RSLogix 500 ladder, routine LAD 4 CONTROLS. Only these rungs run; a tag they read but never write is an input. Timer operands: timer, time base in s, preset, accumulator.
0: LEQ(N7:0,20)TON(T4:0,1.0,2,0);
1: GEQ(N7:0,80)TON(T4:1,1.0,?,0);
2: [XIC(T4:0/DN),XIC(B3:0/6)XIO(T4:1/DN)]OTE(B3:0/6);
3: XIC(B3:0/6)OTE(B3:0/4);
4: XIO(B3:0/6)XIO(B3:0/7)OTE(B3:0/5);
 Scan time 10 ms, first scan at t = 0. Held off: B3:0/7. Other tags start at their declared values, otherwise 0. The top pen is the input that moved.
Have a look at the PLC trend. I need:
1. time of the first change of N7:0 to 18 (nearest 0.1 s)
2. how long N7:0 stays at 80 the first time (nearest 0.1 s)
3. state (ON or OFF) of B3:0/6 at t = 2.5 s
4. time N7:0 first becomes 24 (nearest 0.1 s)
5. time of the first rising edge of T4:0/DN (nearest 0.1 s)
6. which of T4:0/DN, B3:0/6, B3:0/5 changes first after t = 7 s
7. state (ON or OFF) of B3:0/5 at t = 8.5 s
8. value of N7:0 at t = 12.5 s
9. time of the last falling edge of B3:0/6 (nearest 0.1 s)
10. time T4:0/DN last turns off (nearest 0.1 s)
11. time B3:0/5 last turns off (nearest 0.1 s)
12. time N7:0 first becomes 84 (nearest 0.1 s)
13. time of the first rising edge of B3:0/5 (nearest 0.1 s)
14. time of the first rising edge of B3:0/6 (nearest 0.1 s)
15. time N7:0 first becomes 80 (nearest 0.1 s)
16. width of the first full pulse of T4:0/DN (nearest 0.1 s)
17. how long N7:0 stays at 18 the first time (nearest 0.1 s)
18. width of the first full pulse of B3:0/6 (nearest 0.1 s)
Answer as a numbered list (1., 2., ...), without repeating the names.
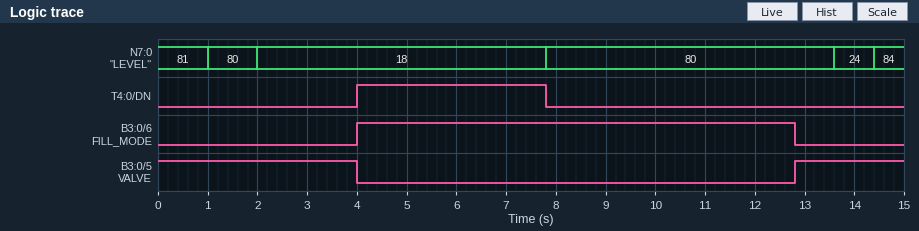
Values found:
1. 2.0 s
2. 1.0 s
3. OFF
4. 13.6 s
5. 4.0 s
6. T4:0/DN
7. OFF
8. 80
9. 12.8 s
10. 7.8 s
11. 4.0 s
12. 14.4 s
13. 12.8 s
14. 4.0 s
15. 1.0 s
16. 3.8 s
17. 5.8 s
18. 8.8 s
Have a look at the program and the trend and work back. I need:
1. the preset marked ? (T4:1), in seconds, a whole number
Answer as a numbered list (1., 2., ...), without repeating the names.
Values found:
1. 5 s
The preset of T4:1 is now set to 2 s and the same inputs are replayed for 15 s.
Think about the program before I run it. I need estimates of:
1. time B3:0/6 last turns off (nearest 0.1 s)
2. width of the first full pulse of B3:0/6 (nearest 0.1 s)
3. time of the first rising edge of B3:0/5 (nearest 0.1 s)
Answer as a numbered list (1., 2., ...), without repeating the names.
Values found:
1. 9.8 s
2. 5.8 s
3. 9.8 s
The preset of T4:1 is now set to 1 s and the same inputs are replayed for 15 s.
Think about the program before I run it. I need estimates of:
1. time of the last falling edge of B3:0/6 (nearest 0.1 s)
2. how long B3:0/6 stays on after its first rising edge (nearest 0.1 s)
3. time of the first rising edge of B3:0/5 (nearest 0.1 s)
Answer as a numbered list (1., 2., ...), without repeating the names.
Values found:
1. 8.8 s
2. 4.8 s
3. 8.8 s
